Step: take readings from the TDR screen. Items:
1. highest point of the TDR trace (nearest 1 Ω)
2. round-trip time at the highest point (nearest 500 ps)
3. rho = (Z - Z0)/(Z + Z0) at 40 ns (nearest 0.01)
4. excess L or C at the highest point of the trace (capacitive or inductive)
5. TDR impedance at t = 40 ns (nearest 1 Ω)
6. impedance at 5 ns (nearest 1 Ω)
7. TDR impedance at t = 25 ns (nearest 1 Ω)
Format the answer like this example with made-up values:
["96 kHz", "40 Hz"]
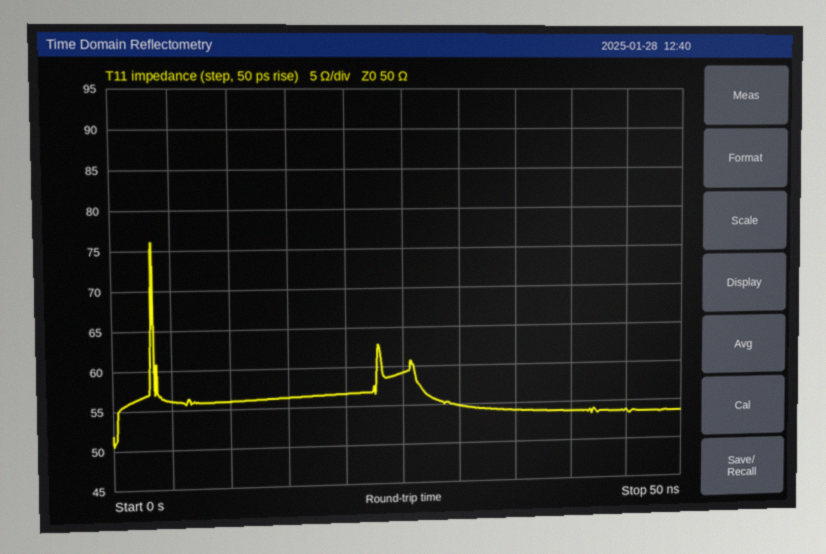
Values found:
["76 Ω", "3.5 ns", "+0.04", "inductive", "54 Ω", "56 Ω", "59 Ω"]
